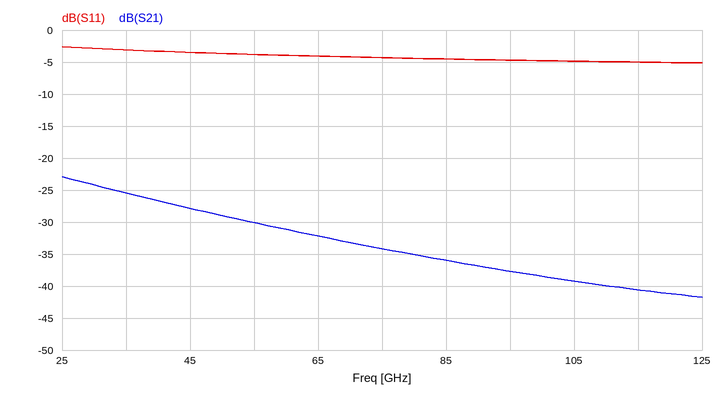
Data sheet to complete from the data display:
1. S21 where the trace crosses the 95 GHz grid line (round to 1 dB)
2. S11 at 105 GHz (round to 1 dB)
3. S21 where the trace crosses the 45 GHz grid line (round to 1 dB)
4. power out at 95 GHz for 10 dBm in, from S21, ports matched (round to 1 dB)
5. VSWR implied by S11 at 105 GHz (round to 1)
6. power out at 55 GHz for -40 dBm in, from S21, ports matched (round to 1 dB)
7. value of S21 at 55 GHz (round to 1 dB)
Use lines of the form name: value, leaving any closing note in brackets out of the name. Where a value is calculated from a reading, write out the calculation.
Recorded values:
S21 where the trace crosses the 95 GHz grid line: -38 dB
S11 at 105 GHz: -5 dB
S21 where the trace crosses the 45 GHz grid line: -28 dB
power out at 95 GHz for 10 dBm in, from S21, ports matched: 10 dBm + (-38 dB) = -28 dBm
VSWR implied by S11 at 105 GHz: |Γ| = 10^(-5/20) = 0.5623; VSWR = (1 + 0.5623)/(1 − 0.5623) ≈ 4
power out at 55 GHz for -40 dBm in, from S21, ports matched: -40 dBm + (-30 dB) = -70 dBm
value of S21 at 55 GHz: -30 dB
